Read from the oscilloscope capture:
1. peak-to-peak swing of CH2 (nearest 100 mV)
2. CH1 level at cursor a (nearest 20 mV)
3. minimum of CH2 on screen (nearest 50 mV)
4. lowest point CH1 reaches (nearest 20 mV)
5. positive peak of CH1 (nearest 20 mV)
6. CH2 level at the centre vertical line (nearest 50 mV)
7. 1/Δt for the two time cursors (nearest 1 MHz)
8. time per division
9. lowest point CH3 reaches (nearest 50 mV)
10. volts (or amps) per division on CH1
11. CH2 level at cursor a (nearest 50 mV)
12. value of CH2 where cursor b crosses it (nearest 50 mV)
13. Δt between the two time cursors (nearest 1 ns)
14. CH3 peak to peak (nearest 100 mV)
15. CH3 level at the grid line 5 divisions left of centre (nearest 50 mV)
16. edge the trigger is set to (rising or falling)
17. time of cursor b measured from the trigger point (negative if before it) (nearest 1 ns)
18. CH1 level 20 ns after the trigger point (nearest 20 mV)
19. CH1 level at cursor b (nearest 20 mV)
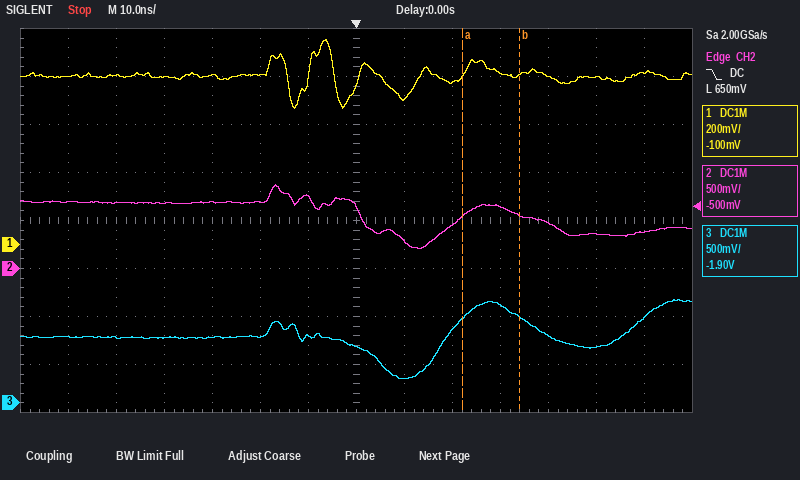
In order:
700 mV
700 mV
200 mV
560 mV
860 mV
650 mV
83 MHz
10 ns
250 mV
200 mV
550 mV
550 mV
12 ns
800 mV
700 mV
falling
+34 ns
680 mV
700 mV
